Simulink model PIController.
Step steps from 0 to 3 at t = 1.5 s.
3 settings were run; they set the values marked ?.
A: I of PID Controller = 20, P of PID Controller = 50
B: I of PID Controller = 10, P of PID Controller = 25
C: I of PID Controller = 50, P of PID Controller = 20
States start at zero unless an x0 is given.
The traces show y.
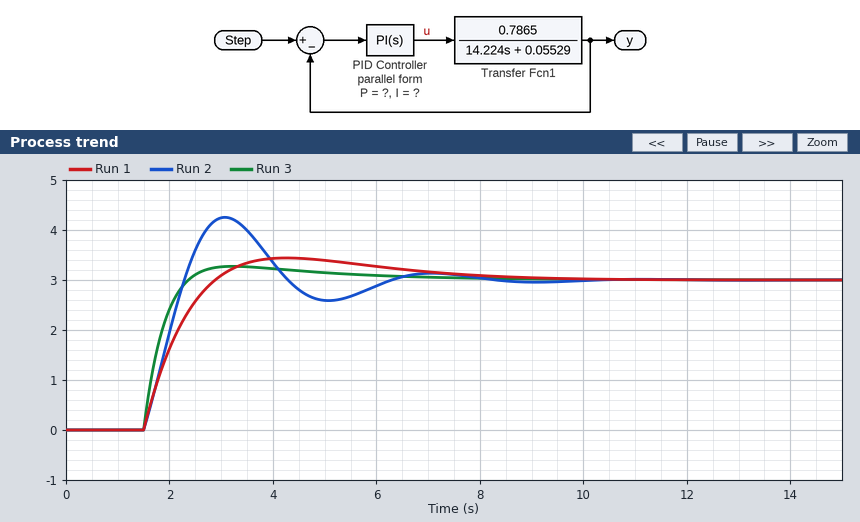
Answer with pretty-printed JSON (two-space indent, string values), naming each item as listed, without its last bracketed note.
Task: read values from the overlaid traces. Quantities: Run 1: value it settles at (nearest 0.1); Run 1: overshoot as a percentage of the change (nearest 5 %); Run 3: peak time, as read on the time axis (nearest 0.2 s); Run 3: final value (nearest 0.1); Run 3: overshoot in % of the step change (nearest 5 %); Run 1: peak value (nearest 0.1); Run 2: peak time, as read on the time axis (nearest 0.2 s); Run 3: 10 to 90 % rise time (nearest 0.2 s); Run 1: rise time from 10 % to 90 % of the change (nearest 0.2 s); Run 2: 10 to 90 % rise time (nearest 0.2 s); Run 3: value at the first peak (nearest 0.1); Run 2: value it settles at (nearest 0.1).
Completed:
{
  "Run 1: value it settles at": "3.0",
  "Run 1: overshoot as a percentage of the change": "15 %",
  "Run 3: peak time, as read on the time axis": "3.2 s",
  "Run 3: final value": "3.0",
  "Run 3: overshoot in % of the step change": "10 %",
  "Run 1: peak value": "3.4",
  "Run 2: peak time, as read on the time axis": "3.0 s",
  "Run 3: 10 to 90 % rise time": "0.6 s",
  "Run 1: rise time from 10 % to 90 % of the change": "1.0 s",
  "Run 2: 10 to 90 % rise time": "0.6 s",
  "Run 3: value at the first peak": "3.3",
  "Run 2: value it settles at": "3.0"
}
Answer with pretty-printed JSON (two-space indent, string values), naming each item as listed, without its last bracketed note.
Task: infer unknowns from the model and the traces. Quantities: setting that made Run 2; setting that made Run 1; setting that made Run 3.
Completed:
{
  "setting that made Run 2": "C",
  "setting that made Run 1": "B",
  "setting that made Run 3": "A"
}
